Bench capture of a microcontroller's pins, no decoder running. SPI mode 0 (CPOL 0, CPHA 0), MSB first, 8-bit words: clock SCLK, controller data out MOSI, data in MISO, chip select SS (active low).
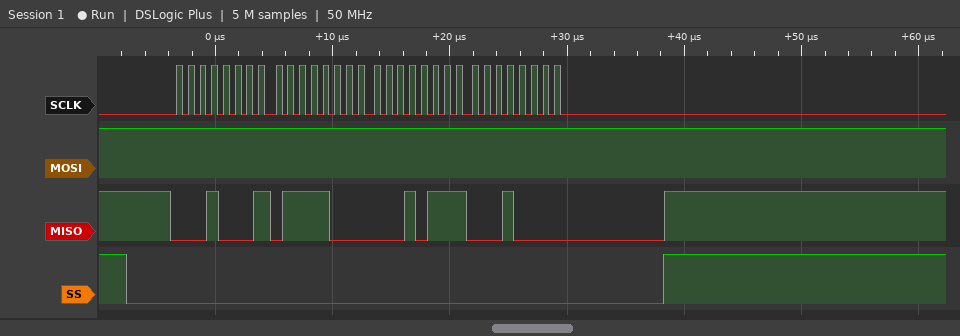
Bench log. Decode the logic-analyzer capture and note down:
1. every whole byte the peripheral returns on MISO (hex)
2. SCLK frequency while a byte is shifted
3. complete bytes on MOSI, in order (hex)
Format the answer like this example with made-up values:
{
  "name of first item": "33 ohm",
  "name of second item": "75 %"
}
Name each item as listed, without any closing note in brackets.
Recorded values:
{
  "every whole byte the peripheral returns on MISO": "0x11 0x78 0x17 0x10",
  "SCLK frequency while a byte is shifted": "1 MHz",
  "complete bytes on MOSI, in order": "0xFF 0xFF 0xFF 0xFF"
}
